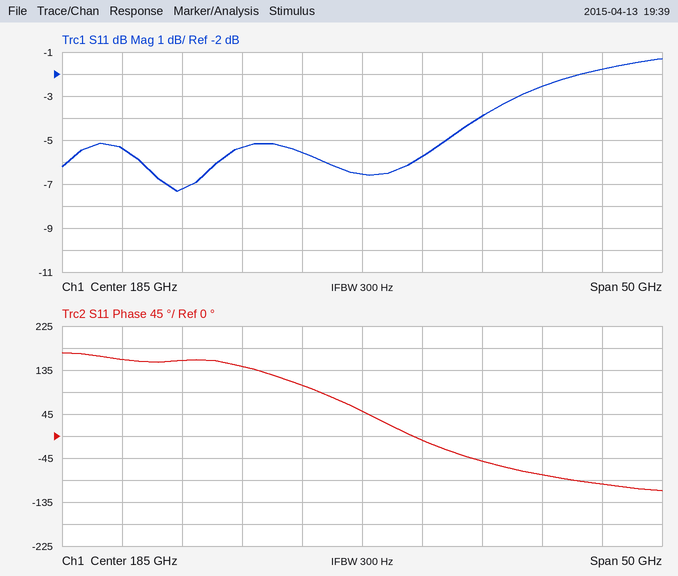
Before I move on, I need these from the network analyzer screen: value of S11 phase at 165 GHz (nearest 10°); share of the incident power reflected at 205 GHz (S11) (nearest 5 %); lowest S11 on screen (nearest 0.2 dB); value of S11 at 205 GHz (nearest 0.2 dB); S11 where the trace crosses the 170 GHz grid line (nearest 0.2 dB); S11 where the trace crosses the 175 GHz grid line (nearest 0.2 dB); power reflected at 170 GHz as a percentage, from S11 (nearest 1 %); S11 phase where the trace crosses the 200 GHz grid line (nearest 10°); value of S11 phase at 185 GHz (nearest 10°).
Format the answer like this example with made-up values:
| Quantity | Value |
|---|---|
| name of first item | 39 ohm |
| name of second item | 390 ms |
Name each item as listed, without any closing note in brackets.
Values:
| Quantity | Value |
|---|---|
| value of S11 phase at 165 GHz | 160° |
| share of the incident power reflected at 205 GHz (S11) | 65 % |
| lowest S11 on screen | -7.4 dB |
| value of S11 at 205 GHz | -1.8 dB |
| S11 where the trace crosses the 170 GHz grid line | -7.2 dB |
| S11 where the trace crosses the 175 GHz grid line | -5.4 dB |
| power reflected at 170 GHz as a percentage, from S11 | 19 % |
| S11 phase where the trace crosses the 200 GHz grid line | -80° |
| value of S11 phase at 185 GHz | 50° |
